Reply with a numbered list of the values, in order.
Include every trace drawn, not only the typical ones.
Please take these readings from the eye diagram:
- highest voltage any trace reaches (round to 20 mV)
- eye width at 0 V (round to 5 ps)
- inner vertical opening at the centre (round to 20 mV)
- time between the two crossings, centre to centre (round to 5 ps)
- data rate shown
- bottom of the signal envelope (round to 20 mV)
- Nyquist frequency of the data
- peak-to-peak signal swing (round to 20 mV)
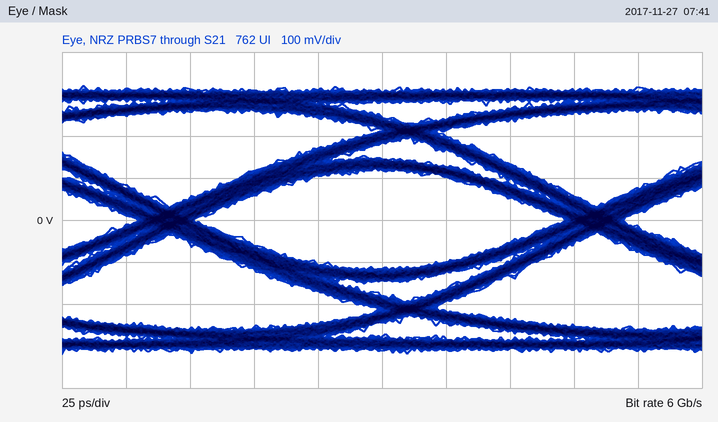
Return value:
1. 320 mV
2. 145 ps
3. 240 mV
4. 165 ps
5. 6 Gb/s
6. -320 mV
7. 3 GHz
8. 640 mV
